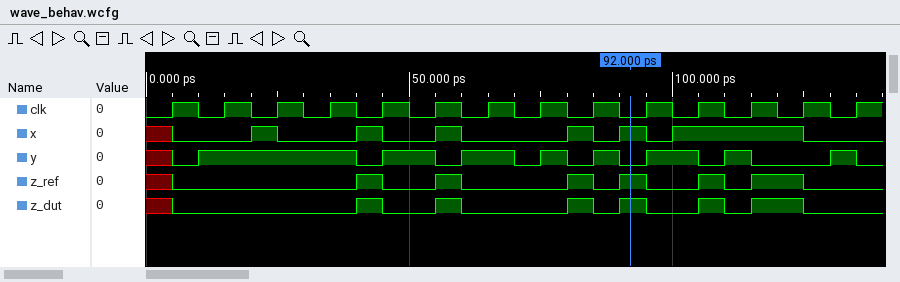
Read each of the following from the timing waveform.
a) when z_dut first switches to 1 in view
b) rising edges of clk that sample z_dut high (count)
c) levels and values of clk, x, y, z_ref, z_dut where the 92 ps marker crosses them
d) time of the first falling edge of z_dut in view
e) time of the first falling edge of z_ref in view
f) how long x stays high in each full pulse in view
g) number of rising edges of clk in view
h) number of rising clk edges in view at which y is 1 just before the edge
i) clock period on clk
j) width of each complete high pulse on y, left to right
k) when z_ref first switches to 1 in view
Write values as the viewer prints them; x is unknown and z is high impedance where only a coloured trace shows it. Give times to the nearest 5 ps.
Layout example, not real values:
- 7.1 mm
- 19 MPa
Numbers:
- 40 ps
- 4
- clk=0, x=1, y=0, z_ref=1, z_dut=1
- 45 ps
- 45 ps
- 5 ps, 5 ps, 5 ps, 5 ps, 5 ps, 25 ps
- 14
- 8
- 10 ps
- 30 ps, 10 ps, 10 ps, 5 ps, 5 ps, 10 ps, 5 ps, 5 ps
- 40 ps
